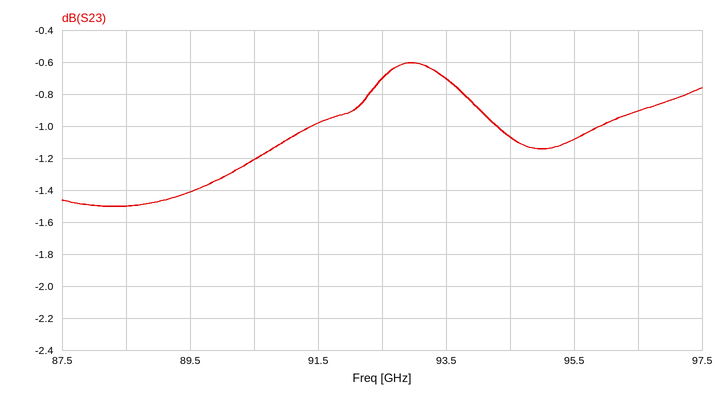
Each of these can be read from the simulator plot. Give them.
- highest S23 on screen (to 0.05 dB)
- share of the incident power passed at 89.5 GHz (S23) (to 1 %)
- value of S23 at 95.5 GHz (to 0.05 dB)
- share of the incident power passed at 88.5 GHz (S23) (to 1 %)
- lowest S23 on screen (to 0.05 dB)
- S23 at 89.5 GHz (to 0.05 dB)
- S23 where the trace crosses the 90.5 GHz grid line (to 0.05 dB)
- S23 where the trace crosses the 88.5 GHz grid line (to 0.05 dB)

-0.60 dB
72 %
-1.10 dB
71 %
-1.50 dB
-1.40 dB
-1.20 dB
-1.50 dB
